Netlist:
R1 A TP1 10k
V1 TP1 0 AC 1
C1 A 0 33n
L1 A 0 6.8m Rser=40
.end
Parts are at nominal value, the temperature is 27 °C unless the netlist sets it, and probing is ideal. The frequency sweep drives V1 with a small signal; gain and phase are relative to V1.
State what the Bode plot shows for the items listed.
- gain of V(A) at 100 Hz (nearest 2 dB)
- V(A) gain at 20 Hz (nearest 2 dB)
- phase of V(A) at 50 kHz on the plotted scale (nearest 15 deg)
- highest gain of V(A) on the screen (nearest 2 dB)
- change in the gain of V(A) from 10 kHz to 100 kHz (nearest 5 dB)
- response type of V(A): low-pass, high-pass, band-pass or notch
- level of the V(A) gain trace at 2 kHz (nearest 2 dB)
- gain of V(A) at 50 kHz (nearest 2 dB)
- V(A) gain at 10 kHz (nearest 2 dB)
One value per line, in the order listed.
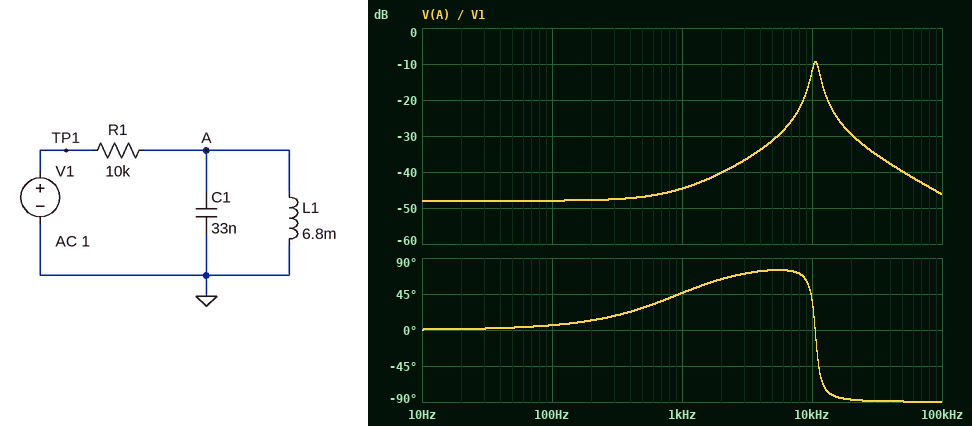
-48 dB
-48 dB
-90 deg
-10 dB
-35 dB
band-pass
-40 dB
-40 dB
-12 dB
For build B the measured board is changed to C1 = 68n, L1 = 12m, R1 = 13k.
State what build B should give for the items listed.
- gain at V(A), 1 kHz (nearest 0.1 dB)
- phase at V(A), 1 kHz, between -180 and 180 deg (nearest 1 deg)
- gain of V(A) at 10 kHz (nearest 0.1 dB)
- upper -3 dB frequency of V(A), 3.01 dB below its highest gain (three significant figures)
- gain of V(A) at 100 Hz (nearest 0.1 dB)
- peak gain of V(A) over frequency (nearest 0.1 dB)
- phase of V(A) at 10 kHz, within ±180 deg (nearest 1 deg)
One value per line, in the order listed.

-43.4 dB
61 deg
-31.7 dB
5.95 kHz
-50.1 dB
-11.9 dB
-87 deg
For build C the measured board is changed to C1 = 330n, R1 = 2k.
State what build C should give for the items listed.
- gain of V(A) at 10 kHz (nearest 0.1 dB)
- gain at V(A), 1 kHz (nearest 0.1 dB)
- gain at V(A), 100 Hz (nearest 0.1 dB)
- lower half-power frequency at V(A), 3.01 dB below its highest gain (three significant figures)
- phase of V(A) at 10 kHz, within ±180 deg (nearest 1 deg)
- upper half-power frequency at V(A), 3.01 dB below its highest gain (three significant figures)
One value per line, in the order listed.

-31.3 dB
-30.1 dB
-34.1 dB
2.84 kHz
-88 deg
4.02 kHz
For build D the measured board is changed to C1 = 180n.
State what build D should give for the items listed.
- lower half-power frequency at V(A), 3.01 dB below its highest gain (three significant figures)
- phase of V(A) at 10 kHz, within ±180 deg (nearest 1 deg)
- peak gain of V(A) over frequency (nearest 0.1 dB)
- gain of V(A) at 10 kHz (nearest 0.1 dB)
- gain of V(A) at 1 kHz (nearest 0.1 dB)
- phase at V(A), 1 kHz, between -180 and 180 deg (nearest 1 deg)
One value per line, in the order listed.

4.07 kHz
-88 deg
-21.1 dB
-39.1 dB
-44.3 dB
44 deg
